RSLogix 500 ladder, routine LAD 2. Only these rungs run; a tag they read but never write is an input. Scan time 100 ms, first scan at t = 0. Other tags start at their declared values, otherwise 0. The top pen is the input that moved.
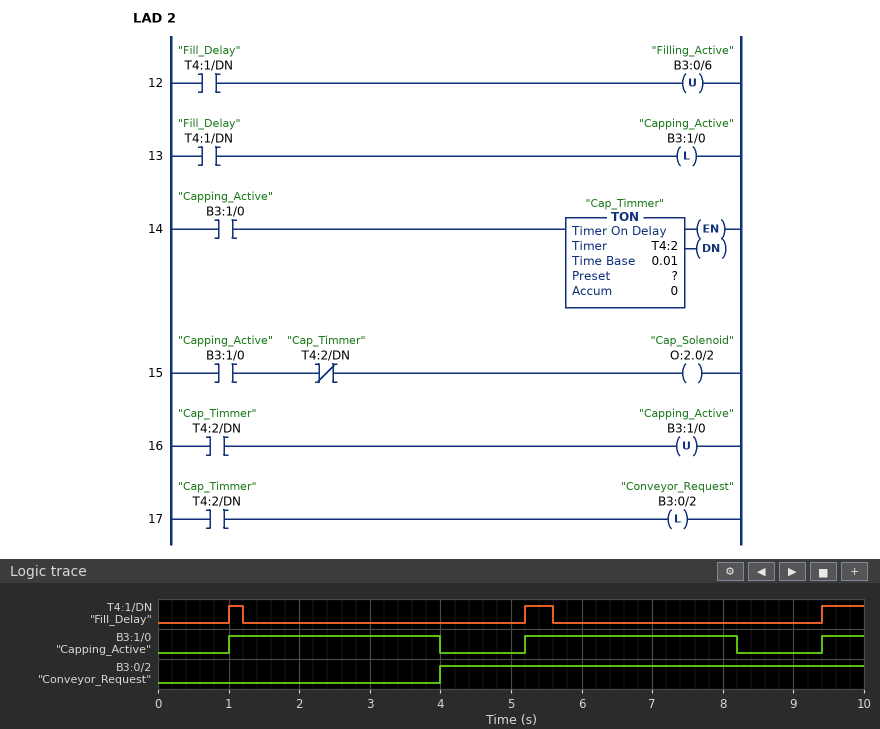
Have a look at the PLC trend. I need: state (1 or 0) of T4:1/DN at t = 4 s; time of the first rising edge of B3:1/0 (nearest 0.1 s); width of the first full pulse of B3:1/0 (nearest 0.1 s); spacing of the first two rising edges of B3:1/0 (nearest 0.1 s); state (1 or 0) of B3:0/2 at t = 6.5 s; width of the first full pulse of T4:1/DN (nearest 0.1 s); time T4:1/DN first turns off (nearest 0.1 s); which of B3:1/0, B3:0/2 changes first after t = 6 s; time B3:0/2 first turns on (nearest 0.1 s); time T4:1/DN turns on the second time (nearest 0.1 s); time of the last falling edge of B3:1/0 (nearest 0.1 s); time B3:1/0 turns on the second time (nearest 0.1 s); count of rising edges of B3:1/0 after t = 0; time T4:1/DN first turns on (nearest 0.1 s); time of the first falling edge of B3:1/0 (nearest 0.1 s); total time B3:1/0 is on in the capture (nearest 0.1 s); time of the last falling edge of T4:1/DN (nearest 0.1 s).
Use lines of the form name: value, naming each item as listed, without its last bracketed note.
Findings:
state (1 or 0) of T4:1/DN at t = 4 s: 0
time of the first rising edge of B3:1/0: 1.0 s
width of the first full pulse of B3:1/0: 3.0 s
spacing of the first two rising edges of B3:1/0: 4.2 s
state (1 or 0) of B3:0/2 at t = 6.5 s: 1
width of the first full pulse of T4:1/DN: 0.2 s
time T4:1/DN first turns off: 1.2 s
which of B3:1/0, B3:0/2 changes first after t = 6 s: B3:1/0
time B3:0/2 first turns on: 4.0 s
time T4:1/DN turns on the second time: 5.2 s
time of the last falling edge of B3:1/0: 8.2 s
time B3:1/0 turns on the second time: 5.2 s
count of rising edges of B3:1/0 after t = 0: 3
time T4:1/DN first turns on: 1.0 s
time of the first falling edge of B3:1/0: 4.0 s
total time B3:1/0 is on in the capture: 6.6 s
time of the last falling edge of T4:1/DN: 5.6 s
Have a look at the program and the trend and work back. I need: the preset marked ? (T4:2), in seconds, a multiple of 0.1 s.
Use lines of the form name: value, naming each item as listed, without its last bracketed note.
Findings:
the preset marked ? (T4:2), in seconds, a multiple of 0.1 s: 3.0 s
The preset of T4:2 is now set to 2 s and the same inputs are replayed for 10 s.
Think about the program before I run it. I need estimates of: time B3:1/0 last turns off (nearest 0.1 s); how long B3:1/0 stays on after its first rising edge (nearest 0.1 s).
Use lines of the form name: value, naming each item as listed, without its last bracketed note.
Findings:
time B3:1/0 last turns off: 7.2 s
how long B3:1/0 stays on after its first rising edge: 2.0 s
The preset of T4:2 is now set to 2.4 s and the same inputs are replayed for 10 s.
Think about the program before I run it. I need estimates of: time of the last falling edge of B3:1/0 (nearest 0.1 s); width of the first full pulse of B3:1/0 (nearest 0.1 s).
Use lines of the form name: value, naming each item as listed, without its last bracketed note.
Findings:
time of the last falling edge of B3:1/0: 7.6 s
width of the first full pulse of B3:1/0: 2.4 s
